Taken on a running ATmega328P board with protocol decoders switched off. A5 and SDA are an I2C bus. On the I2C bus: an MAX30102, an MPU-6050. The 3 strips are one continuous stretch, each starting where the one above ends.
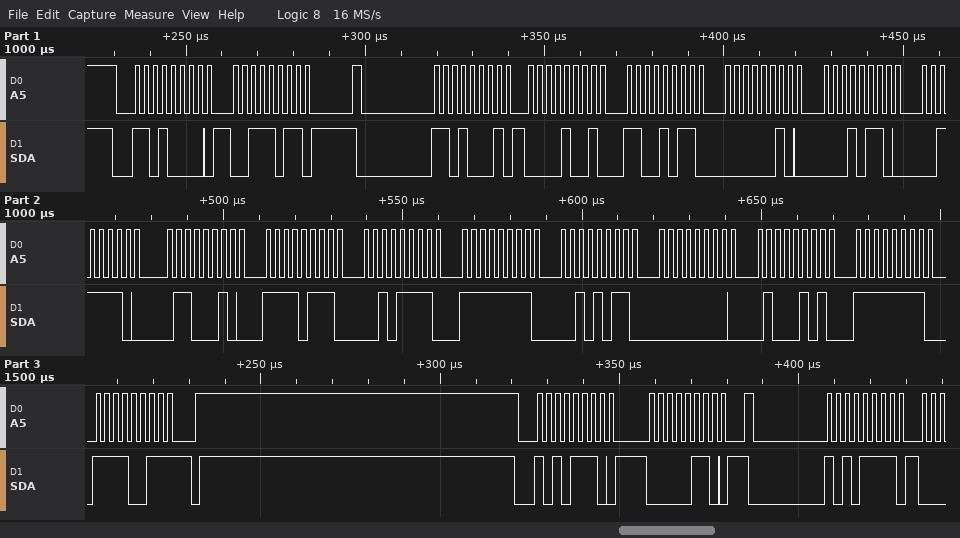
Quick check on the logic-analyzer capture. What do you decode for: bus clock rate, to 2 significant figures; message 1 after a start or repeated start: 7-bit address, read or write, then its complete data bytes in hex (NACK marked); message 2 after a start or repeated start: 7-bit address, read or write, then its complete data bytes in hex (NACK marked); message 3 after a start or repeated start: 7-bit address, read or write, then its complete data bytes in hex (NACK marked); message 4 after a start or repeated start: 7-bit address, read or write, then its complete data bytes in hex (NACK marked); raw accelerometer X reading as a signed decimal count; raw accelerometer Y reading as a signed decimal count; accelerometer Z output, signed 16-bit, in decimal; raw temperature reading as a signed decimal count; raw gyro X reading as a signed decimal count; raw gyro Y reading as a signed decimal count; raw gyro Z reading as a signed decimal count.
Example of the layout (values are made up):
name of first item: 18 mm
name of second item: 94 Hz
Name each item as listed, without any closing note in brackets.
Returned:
bus clock rate, to 2 significant figures: 400 kHz
message 1 after a start or repeated start: 7-bit address, read or write, then its complete data bytes in hex: 0x68 write: 3B
message 2 after a start or repeated start: 7-bit address, read or write, then its complete data bytes in hex: 0x68 read: 09 CB 02 16 3E 62 F7 2F FF 2B 00 45 FF F3 NACK
message 3 after a start or repeated start: 7-bit address, read or write, then its complete data bytes in hex: 0x57 write: 06
message 4 after a start or repeated start: 7-bit address, read or write, then its complete data bytes in hex: 0x57 read
raw accelerometer X reading as a signed decimal count: 2507
raw accelerometer Y reading as a signed decimal count: 534
accelerometer Z output, signed 16-bit, in decimal: 15970
raw temperature reading as a signed decimal count: -2257
raw gyro X reading as a signed decimal count: -213
raw gyro Y reading as a signed decimal count: 69
raw gyro Z reading as a signed decimal count: -13
